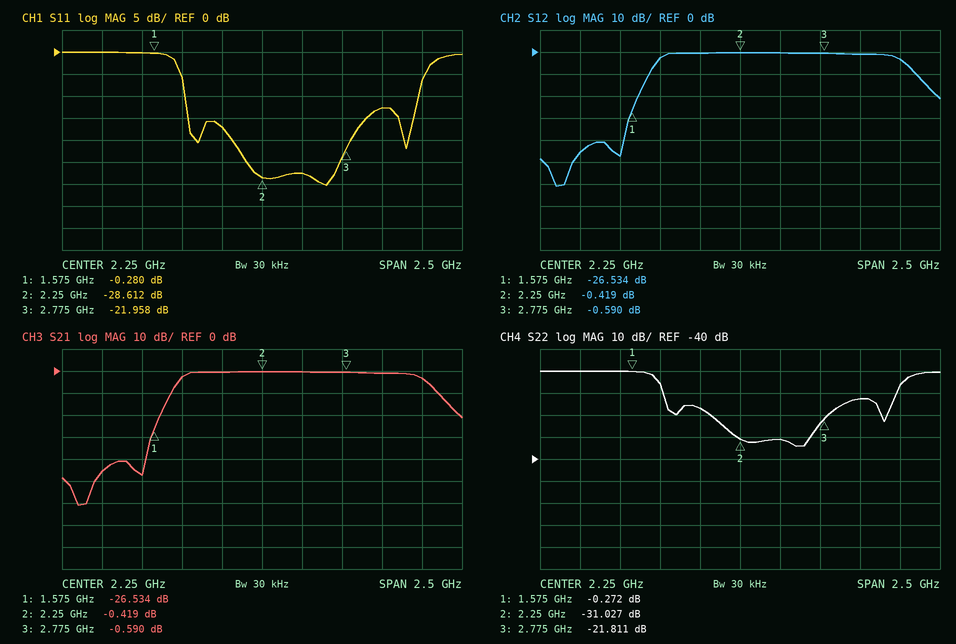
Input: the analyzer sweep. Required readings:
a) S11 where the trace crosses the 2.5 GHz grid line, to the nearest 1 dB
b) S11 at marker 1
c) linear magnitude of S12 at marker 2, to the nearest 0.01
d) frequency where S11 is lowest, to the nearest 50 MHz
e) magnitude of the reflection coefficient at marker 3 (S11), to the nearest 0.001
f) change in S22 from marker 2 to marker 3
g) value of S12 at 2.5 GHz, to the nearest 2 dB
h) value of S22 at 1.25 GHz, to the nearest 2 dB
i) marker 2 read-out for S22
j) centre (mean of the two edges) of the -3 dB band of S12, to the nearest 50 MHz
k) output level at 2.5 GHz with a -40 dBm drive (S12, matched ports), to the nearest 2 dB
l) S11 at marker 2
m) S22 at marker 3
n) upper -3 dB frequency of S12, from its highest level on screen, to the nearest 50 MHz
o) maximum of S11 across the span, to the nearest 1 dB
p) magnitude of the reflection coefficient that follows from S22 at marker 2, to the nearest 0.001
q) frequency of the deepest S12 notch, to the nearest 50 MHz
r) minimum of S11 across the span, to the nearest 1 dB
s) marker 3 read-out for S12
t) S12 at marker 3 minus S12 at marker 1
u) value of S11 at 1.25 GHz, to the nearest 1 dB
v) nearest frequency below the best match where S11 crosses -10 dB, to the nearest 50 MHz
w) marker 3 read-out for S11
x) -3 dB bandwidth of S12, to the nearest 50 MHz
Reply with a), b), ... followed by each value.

a) -28 dB
b) -0.280 dB
c) 0.95
d) 2.65 GHz
e) 0.080
f) 9.216 dB
g) 0 dB
h) 0 dB
i) -31.027 dB
j) 2.50 GHz
k) -40 dBm
l) -28.612 dB
m) -21.811 dB
n) 3.25 GHz
o) 0 dB
p) 0.028
q) 1.10 GHz
r) -30 dB
s) -0.590 dB
t) 25.944 dB
u) 0 dB
v) 1.75 GHz
w) -21.958 dB
x) 1.50 GHz
